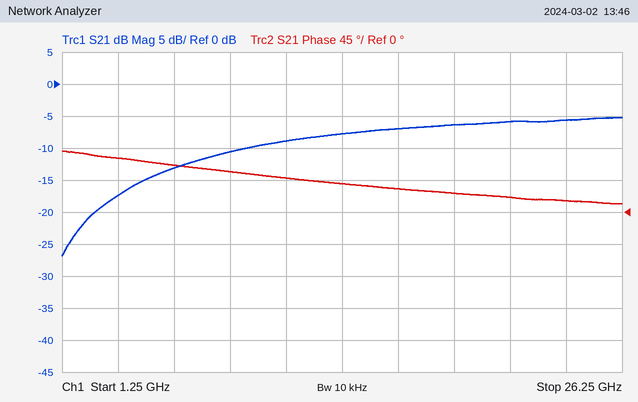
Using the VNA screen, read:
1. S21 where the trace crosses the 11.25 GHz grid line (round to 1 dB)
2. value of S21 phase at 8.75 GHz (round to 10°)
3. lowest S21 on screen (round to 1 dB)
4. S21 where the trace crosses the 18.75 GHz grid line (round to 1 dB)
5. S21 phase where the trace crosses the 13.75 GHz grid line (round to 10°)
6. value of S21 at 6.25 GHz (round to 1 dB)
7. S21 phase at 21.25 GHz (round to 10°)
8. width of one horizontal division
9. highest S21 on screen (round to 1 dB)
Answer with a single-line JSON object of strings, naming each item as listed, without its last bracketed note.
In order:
{"S21 where the trace crosses the 11.25 GHz grid line": "-9 dB", "value of S21 phase at 8.75 GHz": "60°", "lowest S21 on screen": "-27 dB", "S21 where the trace crosses the 18.75 GHz grid line": "-6 dB", "S21 phase where the trace crosses the 13.75 GHz grid line": "40°", "value of S21 at 6.25 GHz": "-13 dB", "S21 phase at 21.25 GHz": "20°", "width of one horizontal division": "2.5 GHz", "highest S21 on screen": "-5 dB"}
